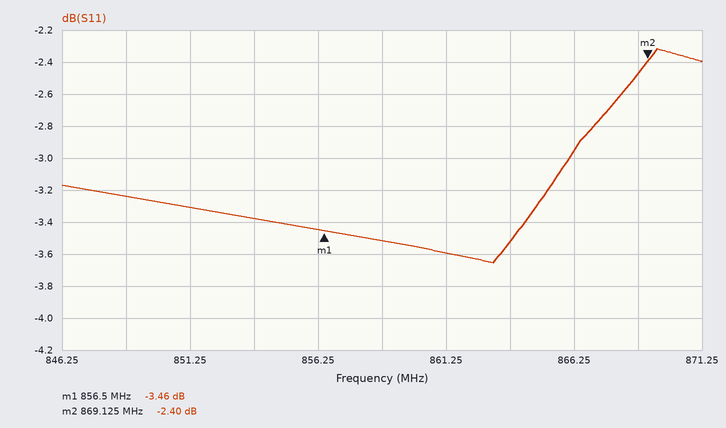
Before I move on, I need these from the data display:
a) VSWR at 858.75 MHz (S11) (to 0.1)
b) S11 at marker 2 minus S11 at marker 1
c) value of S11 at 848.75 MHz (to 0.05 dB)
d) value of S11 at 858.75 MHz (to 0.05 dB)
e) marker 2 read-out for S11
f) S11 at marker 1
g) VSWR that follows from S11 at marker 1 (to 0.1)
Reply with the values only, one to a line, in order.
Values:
5.0
1.06 dB
-3.25 dB
-3.50 dB
-2.40 dB
-3.46 dB
5.1
